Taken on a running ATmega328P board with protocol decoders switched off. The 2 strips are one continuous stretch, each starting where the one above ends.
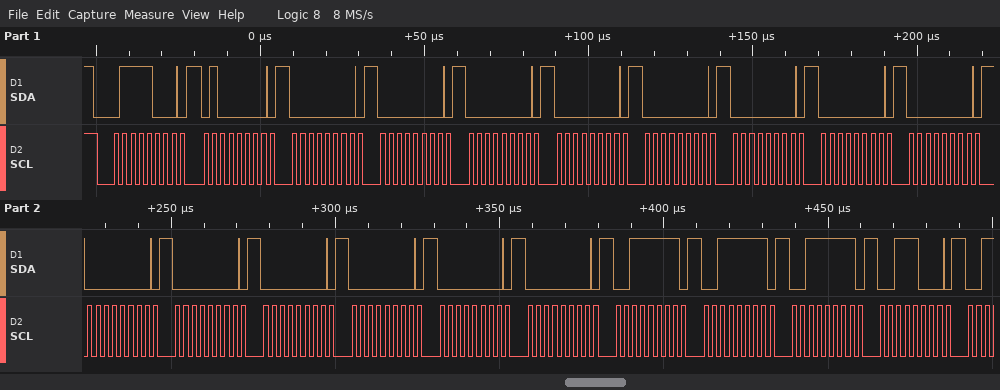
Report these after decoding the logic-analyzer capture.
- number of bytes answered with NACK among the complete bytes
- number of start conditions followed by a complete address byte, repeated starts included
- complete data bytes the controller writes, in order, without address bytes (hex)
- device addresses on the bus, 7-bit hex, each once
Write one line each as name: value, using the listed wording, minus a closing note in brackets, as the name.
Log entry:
number of bytes answered with NACK among the complete bytes: 0
number of start conditions followed by a complete address byte, repeated starts included: 1
complete data bytes the controller writes, in order, without address bytes: 40 00 00 00 00 00 00 00 00 00 00 00 00 00 00 3F 3F 3F 38
device addresses on the bus, 7-bit hex, each once: 0x3C
